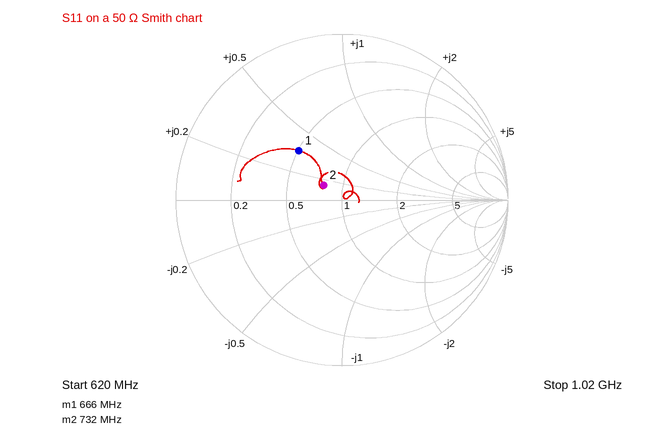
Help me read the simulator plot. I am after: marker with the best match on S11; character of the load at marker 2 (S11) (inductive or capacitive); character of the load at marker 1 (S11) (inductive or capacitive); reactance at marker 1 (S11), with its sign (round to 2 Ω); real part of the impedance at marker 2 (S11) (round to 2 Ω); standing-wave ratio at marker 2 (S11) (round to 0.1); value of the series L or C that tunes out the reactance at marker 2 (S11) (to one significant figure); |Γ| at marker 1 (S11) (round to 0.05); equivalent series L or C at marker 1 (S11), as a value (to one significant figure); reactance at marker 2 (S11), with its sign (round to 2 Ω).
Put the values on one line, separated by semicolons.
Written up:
marker 2; inductive; inductive; +18 Ω; 40 Ω; 1.3; 30 pF; 0.40; 4 nH; +8 Ω
